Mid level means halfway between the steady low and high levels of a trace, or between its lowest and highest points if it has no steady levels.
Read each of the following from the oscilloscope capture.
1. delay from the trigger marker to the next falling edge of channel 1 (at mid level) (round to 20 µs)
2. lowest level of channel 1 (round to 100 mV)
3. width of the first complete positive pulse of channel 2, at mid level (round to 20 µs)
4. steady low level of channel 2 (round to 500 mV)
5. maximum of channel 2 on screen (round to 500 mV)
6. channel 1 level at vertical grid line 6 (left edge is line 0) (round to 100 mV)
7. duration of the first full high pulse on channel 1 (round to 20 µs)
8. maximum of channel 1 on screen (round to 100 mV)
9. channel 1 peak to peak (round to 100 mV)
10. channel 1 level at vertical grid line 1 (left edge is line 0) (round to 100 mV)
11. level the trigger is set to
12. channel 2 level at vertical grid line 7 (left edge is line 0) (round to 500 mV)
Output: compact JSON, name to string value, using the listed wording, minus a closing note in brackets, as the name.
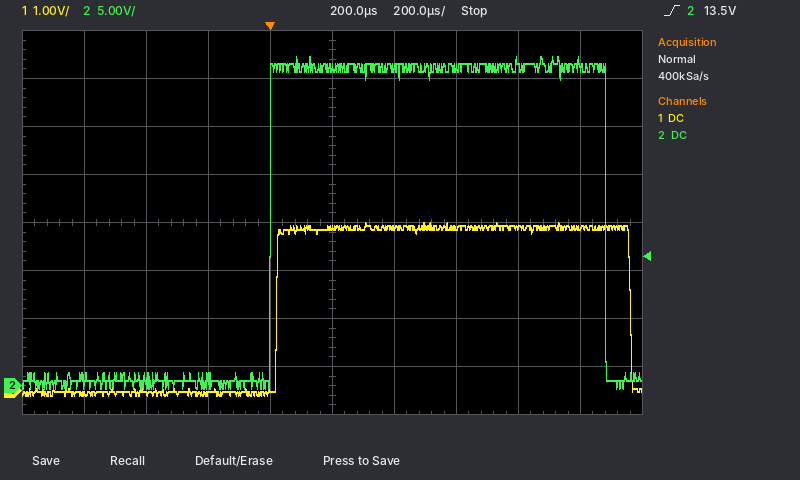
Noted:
{"delay from the trigger marker to the next falling edge of channel 1 (at mid level)": "1.16 ms", "lowest level of channel 1": "-100 mV", "width of the first complete positive pulse of channel 2, at mid level": "1.08 ms", "steady low level of channel 2": "500 mV", "maximum of channel 2 on screen": "34.5 V", "channel 1 level at vertical grid line 6 (left edge is line 0)": "3.4 V", "duration of the first full high pulse on channel 1": "1.14 ms", "maximum of channel 1 on screen": "3.5 V", "channel 1 peak to peak": "3.6 V", "channel 1 level at vertical grid line 1 (left edge is line 0)": "-100 mV", "level the trigger is set to": "13.5 V", "channel 2 level at vertical grid line 7 (left edge is line 0)": "33.0 V"}
